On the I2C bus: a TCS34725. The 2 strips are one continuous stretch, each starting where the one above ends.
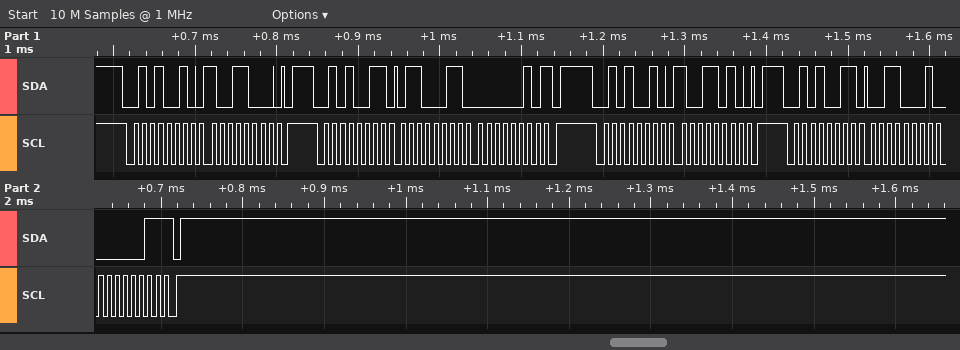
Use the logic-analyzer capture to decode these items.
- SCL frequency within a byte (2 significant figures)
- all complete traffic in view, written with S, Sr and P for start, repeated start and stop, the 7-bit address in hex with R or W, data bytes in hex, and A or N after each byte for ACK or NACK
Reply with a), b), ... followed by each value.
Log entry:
a) 100 kHz
b) S 29W A 98 A P S 29R A 63 A 02 N P S 29W A 9A A P S 29R A 31 A 03 N P
